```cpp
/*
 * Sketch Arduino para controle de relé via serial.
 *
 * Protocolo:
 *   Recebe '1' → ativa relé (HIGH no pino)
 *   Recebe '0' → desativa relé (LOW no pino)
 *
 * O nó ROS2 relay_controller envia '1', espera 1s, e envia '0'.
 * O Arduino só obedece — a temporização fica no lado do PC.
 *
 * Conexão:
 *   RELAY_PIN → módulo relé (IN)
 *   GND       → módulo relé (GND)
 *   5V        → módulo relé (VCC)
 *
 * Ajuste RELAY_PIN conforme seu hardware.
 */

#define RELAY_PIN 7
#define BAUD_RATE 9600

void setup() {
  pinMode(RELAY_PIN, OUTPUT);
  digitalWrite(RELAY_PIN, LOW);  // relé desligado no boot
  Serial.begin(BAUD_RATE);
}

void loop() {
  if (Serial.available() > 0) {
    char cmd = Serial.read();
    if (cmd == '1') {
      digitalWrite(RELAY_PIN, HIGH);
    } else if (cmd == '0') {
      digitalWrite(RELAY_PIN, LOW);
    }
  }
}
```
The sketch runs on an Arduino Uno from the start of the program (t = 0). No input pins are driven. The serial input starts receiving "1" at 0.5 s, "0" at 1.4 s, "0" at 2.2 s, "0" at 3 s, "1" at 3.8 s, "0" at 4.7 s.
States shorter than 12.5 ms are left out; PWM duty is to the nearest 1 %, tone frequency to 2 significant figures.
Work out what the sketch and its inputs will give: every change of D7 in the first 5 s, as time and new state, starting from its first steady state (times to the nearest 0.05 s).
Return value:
0 s low; 0.5 s high; 1.4 s low; 3.8 s high; 4.7 s low
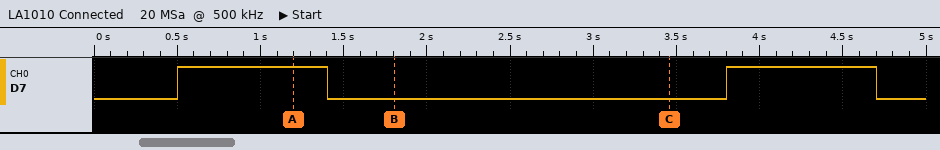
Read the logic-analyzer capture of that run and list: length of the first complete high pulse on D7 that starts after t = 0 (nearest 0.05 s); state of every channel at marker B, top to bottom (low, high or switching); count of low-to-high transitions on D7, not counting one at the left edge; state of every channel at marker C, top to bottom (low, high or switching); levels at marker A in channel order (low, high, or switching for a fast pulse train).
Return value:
0.90 s
D7 low
2
D7 low
D7 high
